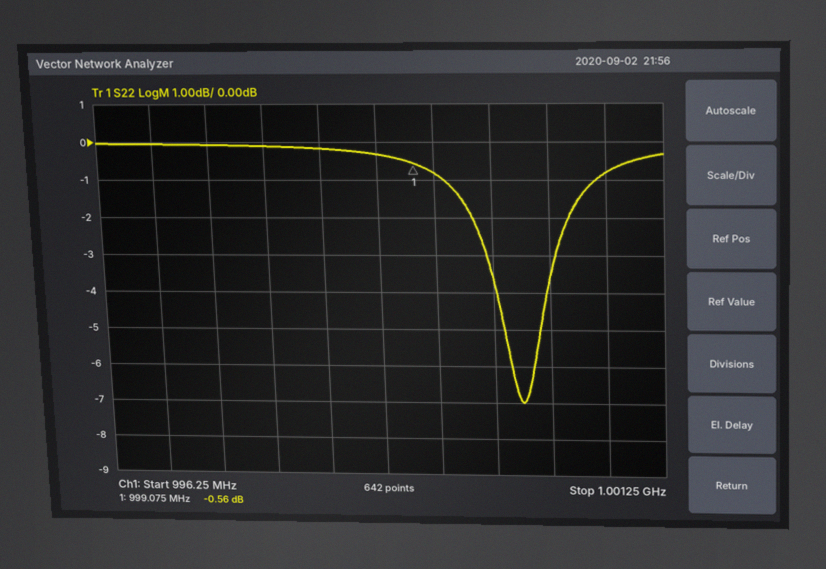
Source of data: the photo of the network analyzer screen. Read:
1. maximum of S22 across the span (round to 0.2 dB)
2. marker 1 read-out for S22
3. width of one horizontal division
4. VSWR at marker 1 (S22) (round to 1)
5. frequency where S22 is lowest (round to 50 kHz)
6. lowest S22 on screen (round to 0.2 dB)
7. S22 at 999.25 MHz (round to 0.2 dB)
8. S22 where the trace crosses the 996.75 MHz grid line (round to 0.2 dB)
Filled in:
0.0 dB
-0.56 dB
500 kHz
31
1.00000 GHz
-7.0 dB
-0.8 dB
0.0 dB
